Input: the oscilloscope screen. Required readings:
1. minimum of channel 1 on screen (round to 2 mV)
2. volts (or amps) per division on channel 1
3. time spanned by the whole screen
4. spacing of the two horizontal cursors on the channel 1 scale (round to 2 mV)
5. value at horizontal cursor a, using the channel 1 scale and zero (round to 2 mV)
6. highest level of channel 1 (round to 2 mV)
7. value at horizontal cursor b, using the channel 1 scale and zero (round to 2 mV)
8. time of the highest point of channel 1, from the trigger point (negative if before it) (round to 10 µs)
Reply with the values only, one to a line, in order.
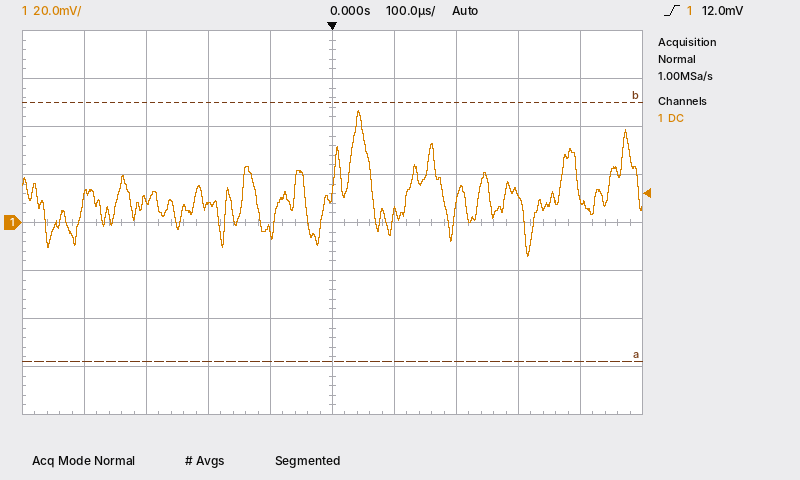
-14 mV
20 mV
1 ms
108 mV
-58 mV
46 mV
50 mV
+40 µs
